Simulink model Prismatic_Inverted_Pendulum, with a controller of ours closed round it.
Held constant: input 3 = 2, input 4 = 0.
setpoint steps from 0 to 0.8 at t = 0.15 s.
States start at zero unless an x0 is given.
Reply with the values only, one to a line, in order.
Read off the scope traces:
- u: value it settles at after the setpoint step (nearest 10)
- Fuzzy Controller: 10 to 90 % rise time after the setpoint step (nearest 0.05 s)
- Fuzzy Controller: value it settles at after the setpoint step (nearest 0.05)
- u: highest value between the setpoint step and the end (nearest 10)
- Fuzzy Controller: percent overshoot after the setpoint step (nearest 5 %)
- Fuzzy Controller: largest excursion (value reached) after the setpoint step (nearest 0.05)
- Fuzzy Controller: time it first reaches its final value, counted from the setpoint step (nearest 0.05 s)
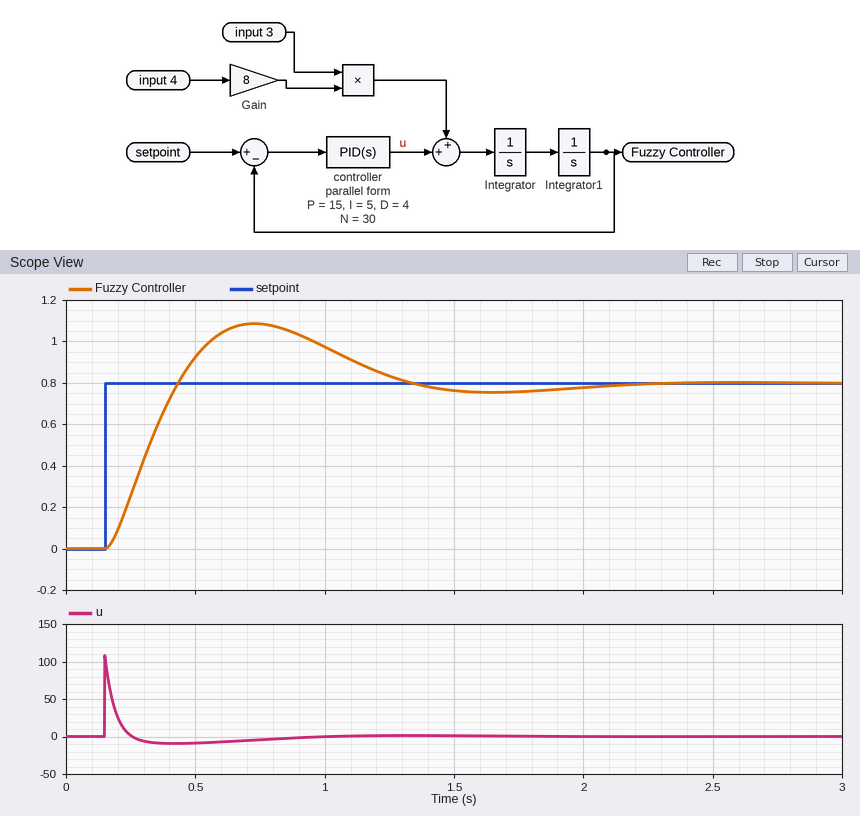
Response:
0
0.20 s
0.80
110
35 %
1.10
0.30 s
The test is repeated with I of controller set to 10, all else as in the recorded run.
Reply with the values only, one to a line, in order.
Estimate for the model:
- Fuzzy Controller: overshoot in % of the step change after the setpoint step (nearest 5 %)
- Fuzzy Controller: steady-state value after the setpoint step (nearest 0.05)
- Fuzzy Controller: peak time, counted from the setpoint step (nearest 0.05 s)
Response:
40 %
0.80
0.60 s
